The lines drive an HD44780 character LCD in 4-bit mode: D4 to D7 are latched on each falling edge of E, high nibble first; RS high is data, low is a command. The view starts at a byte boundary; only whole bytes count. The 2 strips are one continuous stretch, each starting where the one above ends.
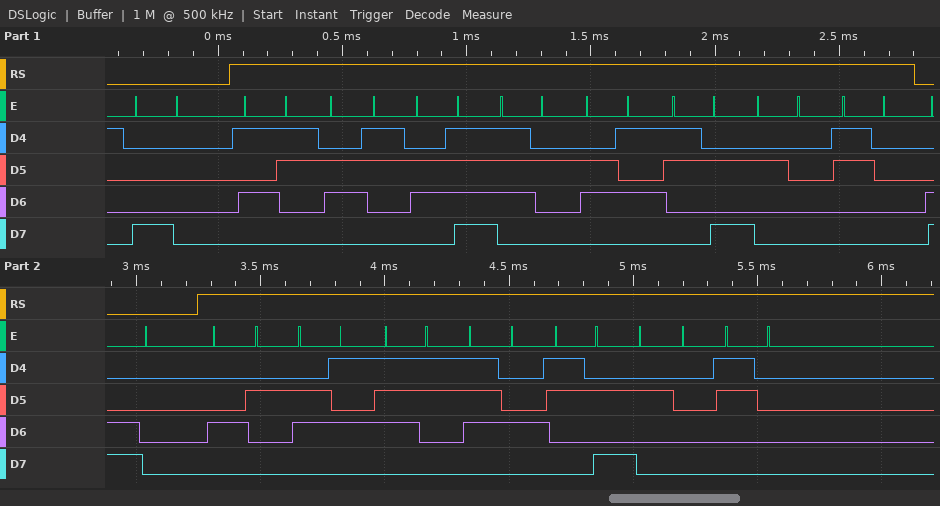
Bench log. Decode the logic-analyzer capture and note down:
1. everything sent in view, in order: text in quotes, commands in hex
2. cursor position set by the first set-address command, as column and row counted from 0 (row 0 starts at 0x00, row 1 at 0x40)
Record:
0x80 "Score: 0" 0xC0 "Best: 0"
column 0, row 0
